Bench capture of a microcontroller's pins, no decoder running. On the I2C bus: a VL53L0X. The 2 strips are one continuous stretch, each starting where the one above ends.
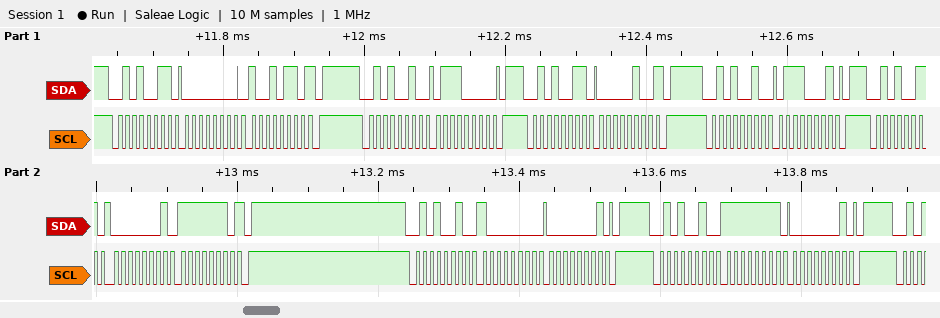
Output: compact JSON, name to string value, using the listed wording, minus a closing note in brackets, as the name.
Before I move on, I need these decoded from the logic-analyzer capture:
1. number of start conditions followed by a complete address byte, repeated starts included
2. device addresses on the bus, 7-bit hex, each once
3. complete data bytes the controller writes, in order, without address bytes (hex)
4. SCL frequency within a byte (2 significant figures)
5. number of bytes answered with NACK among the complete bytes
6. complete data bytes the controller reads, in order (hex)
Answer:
{"number of start conditions followed by a complete address byte, repeated starts included": "7", "device addresses on the bus, 7-bit hex, each once": "0x29", "complete data bytes the controller writes, in order, without address bytes": "70 71 80 01 FF 01", "SCL frequency within a byte": "100 kHz", "number of bytes answered with NACK among the complete bytes": "3", "complete data bytes the controller reads, in order": "00 96 04 01 FE"}
